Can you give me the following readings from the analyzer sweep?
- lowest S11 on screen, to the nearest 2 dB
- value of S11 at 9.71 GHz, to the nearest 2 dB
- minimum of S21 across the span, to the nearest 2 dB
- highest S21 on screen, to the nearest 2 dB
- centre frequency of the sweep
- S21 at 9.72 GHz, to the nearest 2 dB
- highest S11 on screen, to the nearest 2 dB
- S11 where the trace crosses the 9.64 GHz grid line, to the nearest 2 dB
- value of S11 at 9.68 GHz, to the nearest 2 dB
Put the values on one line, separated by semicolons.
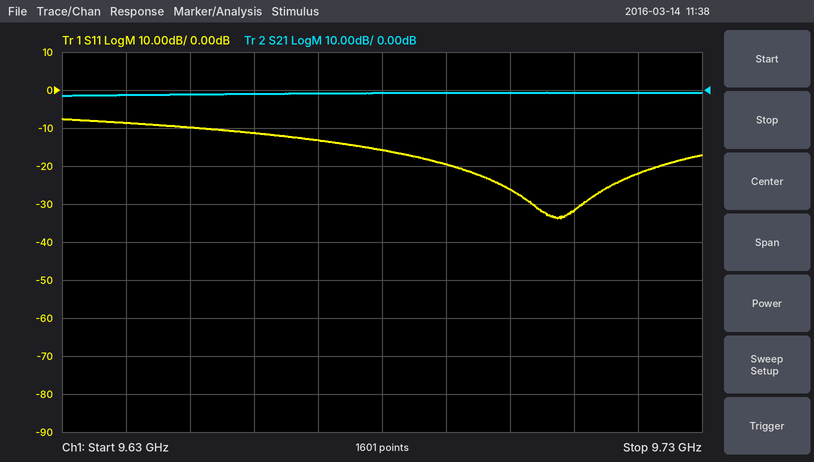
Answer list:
-34 dB; -32 dB; -2 dB; 0 dB; 9.68 GHz; 0 dB; -8 dB; -8 dB; -16 dB
